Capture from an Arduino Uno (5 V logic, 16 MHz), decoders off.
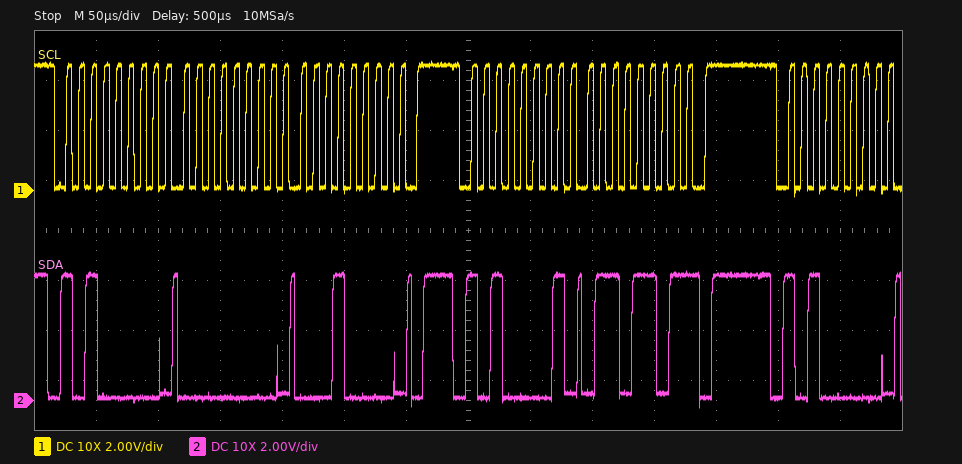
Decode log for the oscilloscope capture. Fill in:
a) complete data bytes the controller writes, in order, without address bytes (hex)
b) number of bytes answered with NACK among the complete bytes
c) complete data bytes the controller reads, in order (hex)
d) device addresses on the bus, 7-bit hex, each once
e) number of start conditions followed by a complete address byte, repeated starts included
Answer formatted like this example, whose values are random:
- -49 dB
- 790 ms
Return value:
- 00 10
- 1
- 6D
- 0x50
- 3
